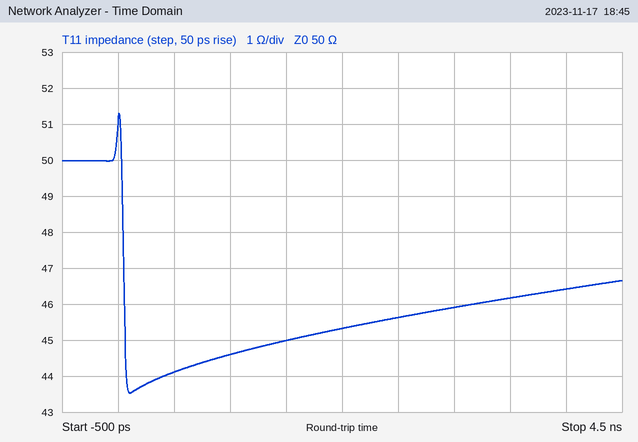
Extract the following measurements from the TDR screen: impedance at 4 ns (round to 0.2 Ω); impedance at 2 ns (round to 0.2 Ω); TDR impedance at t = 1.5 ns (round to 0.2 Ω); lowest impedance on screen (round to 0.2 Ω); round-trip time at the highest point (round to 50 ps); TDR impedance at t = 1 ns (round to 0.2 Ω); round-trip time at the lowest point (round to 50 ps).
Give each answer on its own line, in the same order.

46.4 Ω
45.4 Ω
45.0 Ω
43.6 Ω
0 ps
44.6 Ω
100 ps
